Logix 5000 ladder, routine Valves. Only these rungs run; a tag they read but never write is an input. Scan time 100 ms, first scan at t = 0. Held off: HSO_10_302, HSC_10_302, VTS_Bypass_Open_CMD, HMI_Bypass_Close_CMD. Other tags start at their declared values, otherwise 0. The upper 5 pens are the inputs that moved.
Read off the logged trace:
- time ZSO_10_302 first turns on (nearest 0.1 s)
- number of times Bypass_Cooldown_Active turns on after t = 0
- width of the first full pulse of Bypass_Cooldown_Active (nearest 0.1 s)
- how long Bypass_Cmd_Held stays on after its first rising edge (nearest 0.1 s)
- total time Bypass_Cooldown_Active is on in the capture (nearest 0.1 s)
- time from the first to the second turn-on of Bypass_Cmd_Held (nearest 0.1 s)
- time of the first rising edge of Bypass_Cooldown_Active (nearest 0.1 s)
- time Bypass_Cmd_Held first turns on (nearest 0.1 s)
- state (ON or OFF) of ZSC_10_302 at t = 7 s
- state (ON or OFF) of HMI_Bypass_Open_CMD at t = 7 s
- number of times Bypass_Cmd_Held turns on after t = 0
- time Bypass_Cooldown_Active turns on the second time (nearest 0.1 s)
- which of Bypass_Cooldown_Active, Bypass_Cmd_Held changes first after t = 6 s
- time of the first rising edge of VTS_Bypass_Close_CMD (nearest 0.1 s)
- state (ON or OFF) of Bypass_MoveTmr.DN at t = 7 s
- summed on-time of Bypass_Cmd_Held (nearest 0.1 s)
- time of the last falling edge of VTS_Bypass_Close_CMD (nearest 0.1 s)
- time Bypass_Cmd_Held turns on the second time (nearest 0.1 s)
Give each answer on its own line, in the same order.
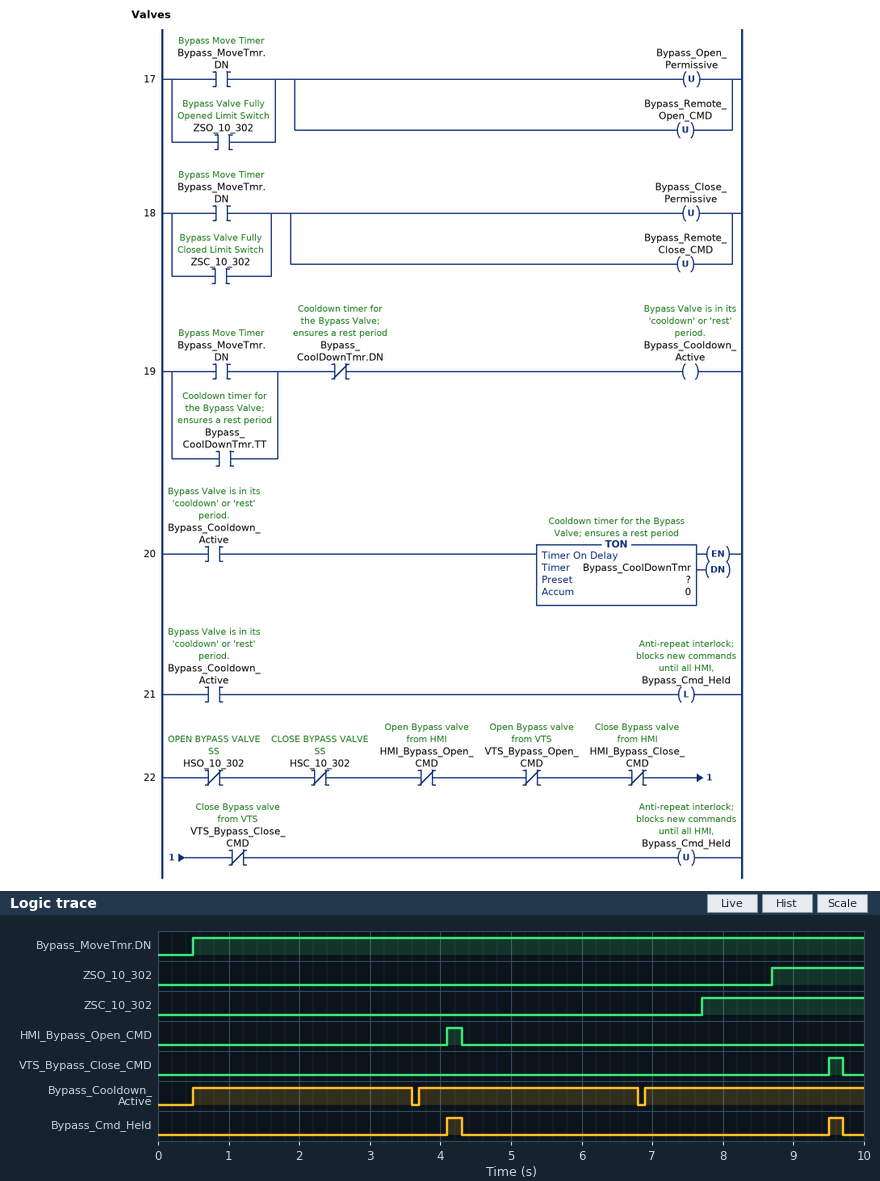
8.7 s
3
3.1 s
0.2 s
9.3 s
5.4 s
0.5 s
4.1 s
OFF
OFF
2
3.7 s
Bypass_Cooldown_Active
9.5 s
ON
0.4 s
9.7 s
9.5 s
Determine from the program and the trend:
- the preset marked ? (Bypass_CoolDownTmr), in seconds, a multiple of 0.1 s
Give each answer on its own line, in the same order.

3.0 s
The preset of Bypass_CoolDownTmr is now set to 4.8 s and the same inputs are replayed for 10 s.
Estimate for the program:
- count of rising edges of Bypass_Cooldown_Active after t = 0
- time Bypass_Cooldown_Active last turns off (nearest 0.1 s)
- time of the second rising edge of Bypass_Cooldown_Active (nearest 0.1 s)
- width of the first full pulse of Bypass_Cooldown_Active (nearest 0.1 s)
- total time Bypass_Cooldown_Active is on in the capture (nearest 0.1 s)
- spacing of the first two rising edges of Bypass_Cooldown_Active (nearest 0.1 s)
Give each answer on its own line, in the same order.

2
5.4 s
5.5 s
4.9 s
9.4 s
5.0 s
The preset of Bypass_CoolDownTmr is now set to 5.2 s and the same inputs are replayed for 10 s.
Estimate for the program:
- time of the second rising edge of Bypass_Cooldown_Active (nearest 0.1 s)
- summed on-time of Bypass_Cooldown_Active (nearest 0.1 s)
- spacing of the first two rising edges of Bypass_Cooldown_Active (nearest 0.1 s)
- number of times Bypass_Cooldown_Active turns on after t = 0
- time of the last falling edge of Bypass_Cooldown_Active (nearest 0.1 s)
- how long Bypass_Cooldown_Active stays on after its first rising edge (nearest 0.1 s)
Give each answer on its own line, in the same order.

5.9 s
9.4 s
5.4 s
2
5.8 s
5.3 s
